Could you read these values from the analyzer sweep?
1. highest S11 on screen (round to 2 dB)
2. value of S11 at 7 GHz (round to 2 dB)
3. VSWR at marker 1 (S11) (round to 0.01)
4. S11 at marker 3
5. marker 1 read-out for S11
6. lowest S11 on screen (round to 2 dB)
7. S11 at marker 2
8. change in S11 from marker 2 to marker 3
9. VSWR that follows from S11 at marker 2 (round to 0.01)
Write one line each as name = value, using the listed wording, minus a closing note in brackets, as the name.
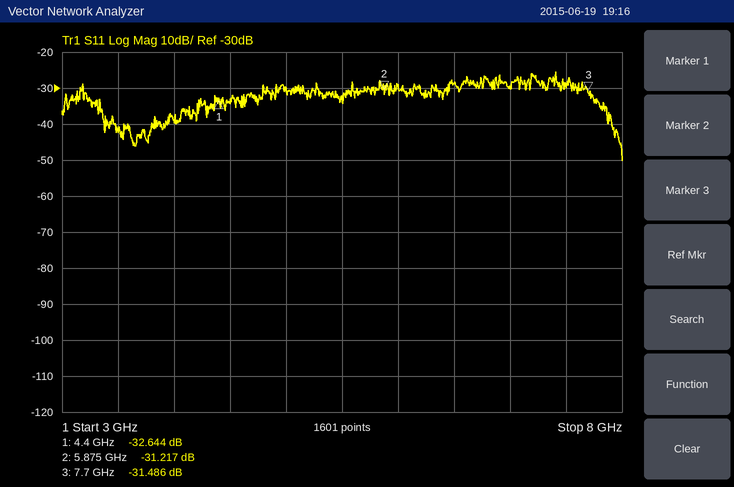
highest S11 on screen = -26 dB
value of S11 at 7 GHz = -30 dB
VSWR at marker 1 (S11) = 1.05
S11 at marker 3 = -31.486 dB
marker 1 read-out for S11 = -32.644 dB
lowest S11 on screen = -50 dB
S11 at marker 2 = -31.217 dB
change in S11 from marker 2 to marker 3 = -0.269 dB
VSWR that follows from S11 at marker 2 = 1.06
